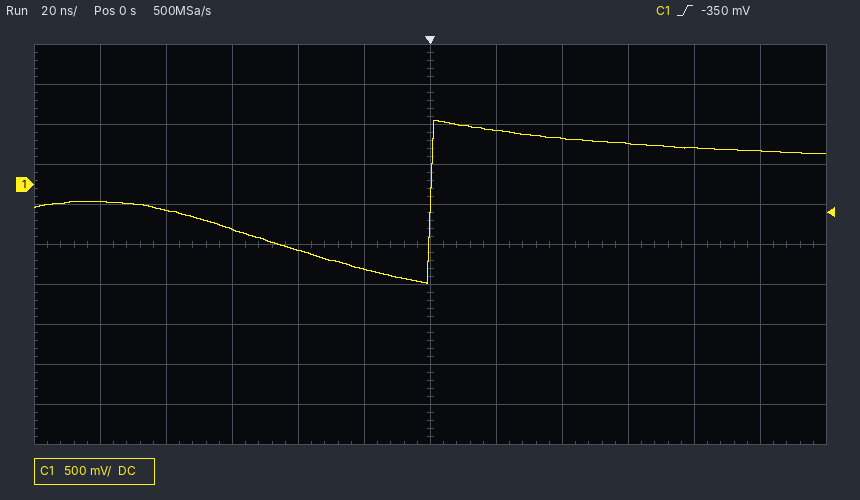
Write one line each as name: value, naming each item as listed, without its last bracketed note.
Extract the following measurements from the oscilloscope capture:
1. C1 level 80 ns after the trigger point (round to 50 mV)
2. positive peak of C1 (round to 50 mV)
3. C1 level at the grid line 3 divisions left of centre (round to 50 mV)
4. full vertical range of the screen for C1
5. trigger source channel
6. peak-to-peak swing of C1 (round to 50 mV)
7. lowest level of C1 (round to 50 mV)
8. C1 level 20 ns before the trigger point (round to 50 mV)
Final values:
C1 level 80 ns after the trigger point: 450 mV
positive peak of C1: 800 mV
C1 level at the grid line 3 divisions left of centre: -550 mV
full vertical range of the screen for C1: 5 V
trigger source channel: C1
peak-to-peak swing of C1: 2.05 V
lowest level of C1: -1.25 V
C1 level 20 ns before the trigger point: -1.05 V
